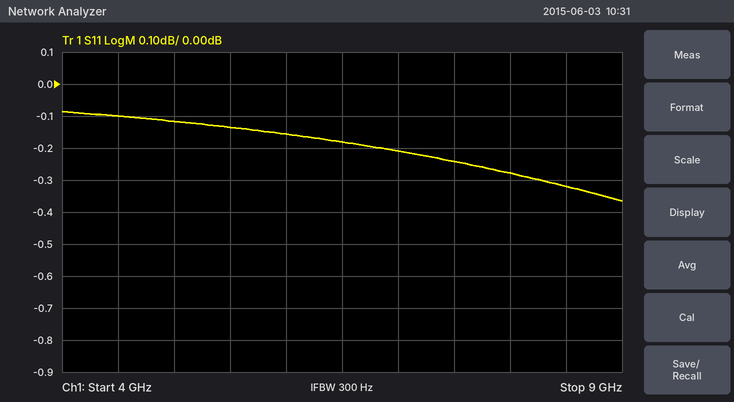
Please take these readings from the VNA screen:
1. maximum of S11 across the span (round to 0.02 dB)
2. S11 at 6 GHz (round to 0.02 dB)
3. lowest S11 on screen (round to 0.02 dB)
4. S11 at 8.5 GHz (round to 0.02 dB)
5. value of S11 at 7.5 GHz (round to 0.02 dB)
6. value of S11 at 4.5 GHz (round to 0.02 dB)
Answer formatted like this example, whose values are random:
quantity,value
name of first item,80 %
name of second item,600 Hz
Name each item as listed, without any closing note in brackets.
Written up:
quantity,value
maximum of S11 across the span,-0.08 dB
S11 at 6 GHz,-0.16 dB
lowest S11 on screen,-0.36 dB
S11 at 8.5 GHz,-0.32 dB
value of S11 at 7.5 GHz,-0.24 dB
value of S11 at 4.5 GHz,-0.10 dB
